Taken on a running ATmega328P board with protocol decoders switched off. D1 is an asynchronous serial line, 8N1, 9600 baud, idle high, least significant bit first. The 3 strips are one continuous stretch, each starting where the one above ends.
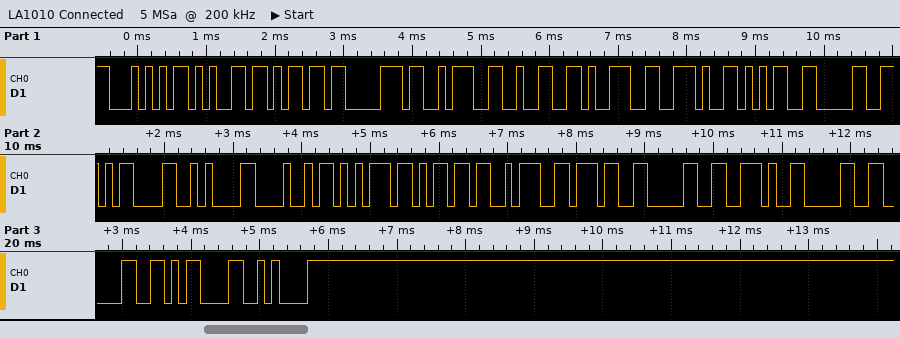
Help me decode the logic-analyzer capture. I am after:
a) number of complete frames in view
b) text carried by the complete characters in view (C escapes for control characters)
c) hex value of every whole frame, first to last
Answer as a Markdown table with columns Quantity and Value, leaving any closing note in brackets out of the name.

| Quantity | Value |
|---|---|
| number of complete frames in view | 23 |
| text carried by the complete characters in view | "Temp:29.50\r\nHum:70.00\r\n" |
| hex value of every whole frame, first to last | 0x54 0x65 0x6D 0x70 0x3A 0x32 0x39 0x2E 0x35 0x30 0x0D 0x0A 0x48 0x75 0x6D 0x3A 0x37 0x30 0x2E 0x30 0x30 0x0D 0x0A |
